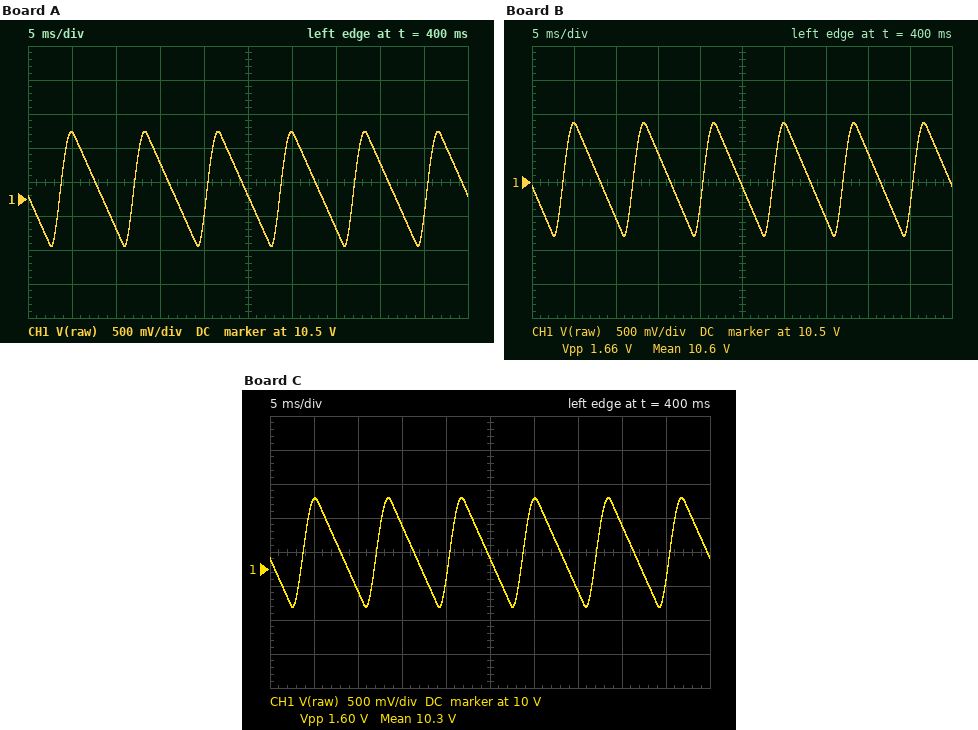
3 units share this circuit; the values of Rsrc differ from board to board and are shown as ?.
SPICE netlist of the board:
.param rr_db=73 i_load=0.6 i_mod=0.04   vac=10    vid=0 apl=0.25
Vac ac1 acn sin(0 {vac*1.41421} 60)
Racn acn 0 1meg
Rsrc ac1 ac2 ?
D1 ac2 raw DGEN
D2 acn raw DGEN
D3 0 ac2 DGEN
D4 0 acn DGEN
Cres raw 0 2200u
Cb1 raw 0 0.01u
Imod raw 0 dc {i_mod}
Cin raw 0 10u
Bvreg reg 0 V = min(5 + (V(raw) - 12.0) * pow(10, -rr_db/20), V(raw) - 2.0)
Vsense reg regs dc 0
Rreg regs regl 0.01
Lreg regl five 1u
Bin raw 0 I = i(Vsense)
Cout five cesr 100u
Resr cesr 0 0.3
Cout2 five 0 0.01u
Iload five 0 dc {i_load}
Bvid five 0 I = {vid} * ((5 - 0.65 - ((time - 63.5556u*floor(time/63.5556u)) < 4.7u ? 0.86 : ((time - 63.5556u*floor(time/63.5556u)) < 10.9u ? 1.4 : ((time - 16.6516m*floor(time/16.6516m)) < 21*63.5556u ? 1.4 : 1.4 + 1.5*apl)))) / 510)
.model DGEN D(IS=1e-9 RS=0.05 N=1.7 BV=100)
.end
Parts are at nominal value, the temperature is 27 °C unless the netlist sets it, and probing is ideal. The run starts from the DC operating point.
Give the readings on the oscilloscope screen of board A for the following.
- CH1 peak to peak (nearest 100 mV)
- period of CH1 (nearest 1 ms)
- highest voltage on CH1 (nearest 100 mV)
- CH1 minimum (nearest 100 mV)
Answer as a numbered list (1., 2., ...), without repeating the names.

1. 1.7 V
2. 8 ms
3. 11.5 V
4. 9.8 V
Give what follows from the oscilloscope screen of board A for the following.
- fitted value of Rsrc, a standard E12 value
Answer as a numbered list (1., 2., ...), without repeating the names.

1. 0.33 Ω
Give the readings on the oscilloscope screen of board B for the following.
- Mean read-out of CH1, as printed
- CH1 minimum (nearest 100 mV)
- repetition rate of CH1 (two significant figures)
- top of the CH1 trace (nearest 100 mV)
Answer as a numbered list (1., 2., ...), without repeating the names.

1. 10.6 V
2. 9.7 V
3. 120 Hz
4. 11.4 V
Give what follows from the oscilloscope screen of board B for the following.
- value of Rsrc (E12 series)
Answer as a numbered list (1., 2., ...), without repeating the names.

1. 0.39 Ω
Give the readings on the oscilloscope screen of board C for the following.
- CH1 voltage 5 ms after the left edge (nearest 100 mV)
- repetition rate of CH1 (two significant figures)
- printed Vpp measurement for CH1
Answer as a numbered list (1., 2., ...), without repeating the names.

1. 11.0 V
2. 120 Hz
3. 1.60 V
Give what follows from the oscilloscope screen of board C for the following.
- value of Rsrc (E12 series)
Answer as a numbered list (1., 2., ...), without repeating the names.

1. 0.56 Ω
